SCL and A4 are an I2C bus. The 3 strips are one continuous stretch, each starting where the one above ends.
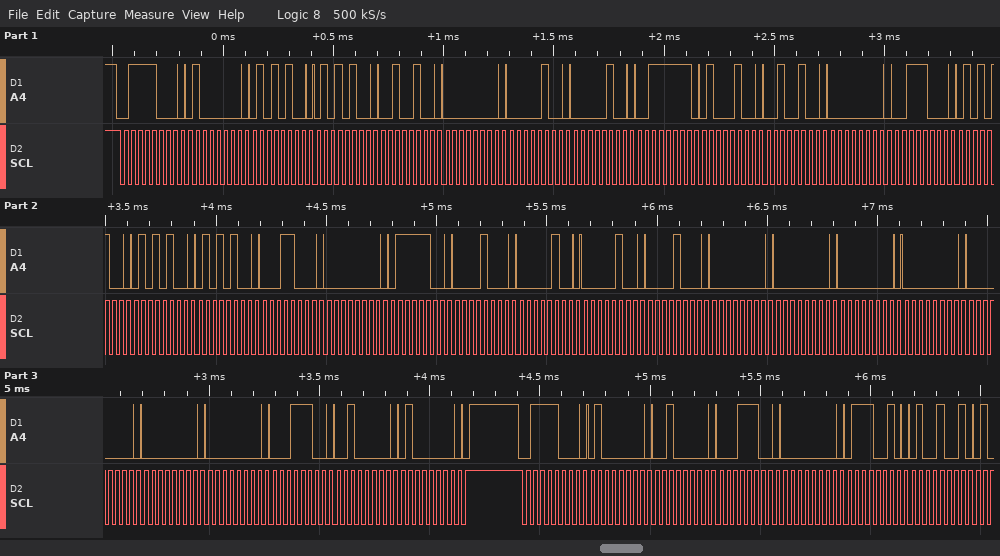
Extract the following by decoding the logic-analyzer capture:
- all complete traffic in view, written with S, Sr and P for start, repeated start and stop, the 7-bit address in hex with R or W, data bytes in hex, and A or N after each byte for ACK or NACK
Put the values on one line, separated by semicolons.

S 3CW A 40 A 54 A 54 A 24 A 00 A 04 A 04 A 3F A 44 A 24 A 00 A 38 A 54 A 54 A 54 A 18 A 00 A 7C A 08 A 04 A 04 A 08 A 00 A 00 A 00 A 00 A 00 A 00 A 00 A 1C A 20 A 40 A P S 3CW A 40 A 20 A 1C A 00 A 72 A 49 A
